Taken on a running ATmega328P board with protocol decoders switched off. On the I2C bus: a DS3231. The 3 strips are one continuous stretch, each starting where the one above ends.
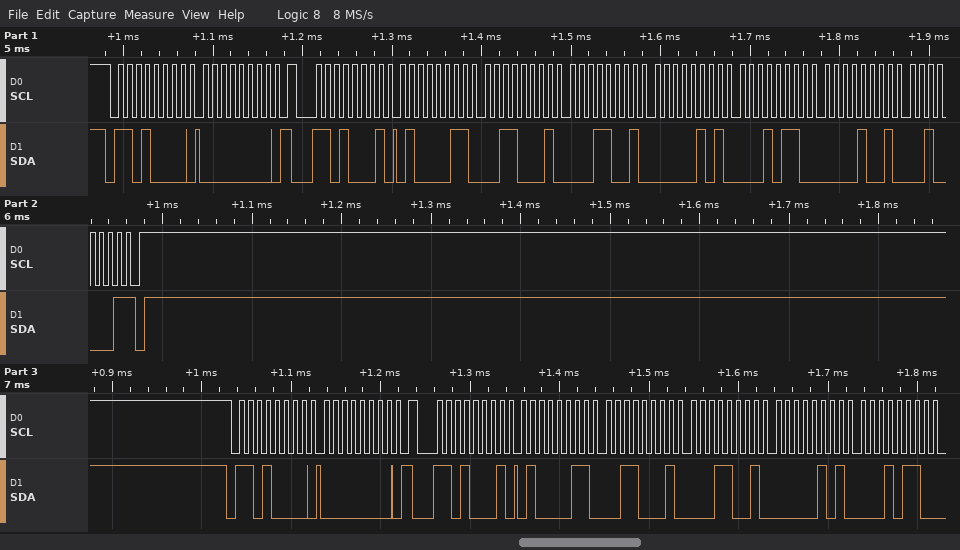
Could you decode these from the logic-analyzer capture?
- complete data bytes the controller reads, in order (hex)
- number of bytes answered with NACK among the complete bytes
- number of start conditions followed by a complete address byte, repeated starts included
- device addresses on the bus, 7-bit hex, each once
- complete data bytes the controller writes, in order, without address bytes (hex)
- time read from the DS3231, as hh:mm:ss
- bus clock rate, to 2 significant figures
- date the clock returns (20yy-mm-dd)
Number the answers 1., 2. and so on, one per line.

1. 43 31 19 05 16 09 21 43 31 19 05 16
2. 1
3. 4
4. 0x68
5. 00 00
6. 19:31:43
7. 100 kHz
8. 2021-09-16
